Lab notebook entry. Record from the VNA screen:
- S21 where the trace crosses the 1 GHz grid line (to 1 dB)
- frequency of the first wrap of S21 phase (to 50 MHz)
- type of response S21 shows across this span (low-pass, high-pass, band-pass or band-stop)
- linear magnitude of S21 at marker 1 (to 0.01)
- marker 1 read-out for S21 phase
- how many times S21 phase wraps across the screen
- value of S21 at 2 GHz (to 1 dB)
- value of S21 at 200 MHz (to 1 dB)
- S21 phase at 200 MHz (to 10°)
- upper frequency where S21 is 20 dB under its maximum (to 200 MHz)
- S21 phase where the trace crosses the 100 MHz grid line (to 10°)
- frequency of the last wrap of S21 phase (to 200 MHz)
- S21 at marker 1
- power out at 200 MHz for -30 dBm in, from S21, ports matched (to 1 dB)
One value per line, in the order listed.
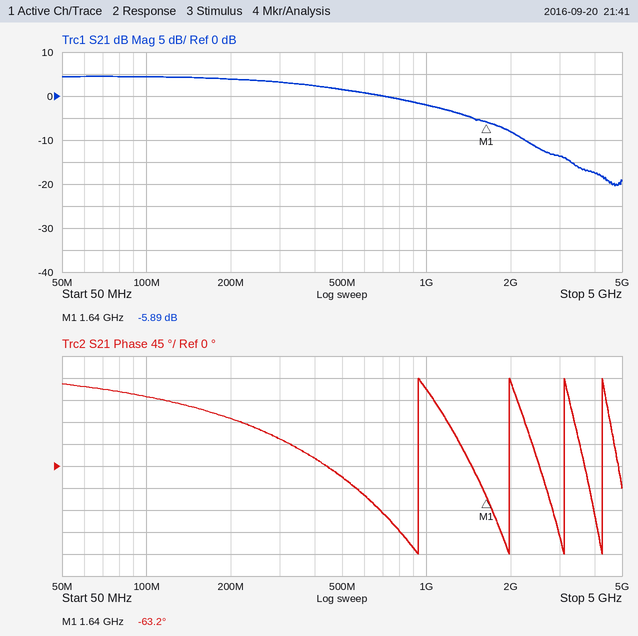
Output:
-2 dB
950 MHz
low-pass
0.51
-63.2°
4
-8 dB
4 dB
100°
3.4 GHz
140°
4.2 GHz
-5.89 dB
-26 dBm
